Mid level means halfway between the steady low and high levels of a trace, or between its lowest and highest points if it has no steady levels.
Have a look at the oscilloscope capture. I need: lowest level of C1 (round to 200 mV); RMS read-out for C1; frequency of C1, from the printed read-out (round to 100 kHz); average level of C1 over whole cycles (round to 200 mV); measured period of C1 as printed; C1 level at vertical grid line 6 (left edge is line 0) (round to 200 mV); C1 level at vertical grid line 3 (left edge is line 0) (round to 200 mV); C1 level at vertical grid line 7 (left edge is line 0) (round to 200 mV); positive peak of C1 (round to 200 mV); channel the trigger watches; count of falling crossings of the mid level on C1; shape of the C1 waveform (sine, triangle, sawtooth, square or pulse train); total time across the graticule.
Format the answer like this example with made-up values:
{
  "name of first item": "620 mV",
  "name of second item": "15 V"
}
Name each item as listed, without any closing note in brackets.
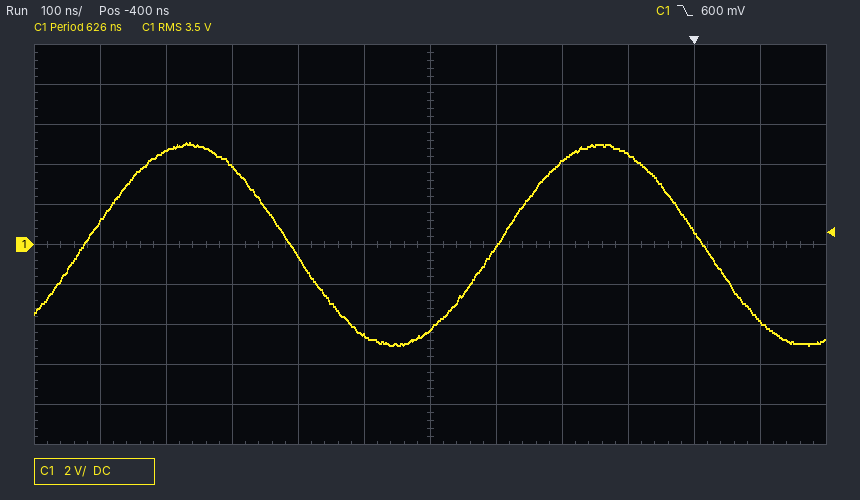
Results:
{
  "lowest level of C1": "-5.0 V",
  "RMS read-out for C1": "3.5 V",
  "frequency of C1, from the printed read-out": "1.6 MHz",
  "average level of C1 over whole cycles": "0.0 V",
  "measured period of C1 as printed": "626 ns",
  "C1 level at vertical grid line 6 (left edge is line 0)": "-4.2 V",
  "C1 level at vertical grid line 3 (left edge is line 0)": "3.8 V",
  "C1 level at vertical grid line 7 (left edge is line 0)": "-200 mV",
  "positive peak of C1": "5.0 V",
  "channel the trigger watches": "C1",
  "count of falling crossings of the mid level on C1": "2",
  "shape of the C1 waveform": "sine",
  "total time across the graticule": "1.2 µs"
}
